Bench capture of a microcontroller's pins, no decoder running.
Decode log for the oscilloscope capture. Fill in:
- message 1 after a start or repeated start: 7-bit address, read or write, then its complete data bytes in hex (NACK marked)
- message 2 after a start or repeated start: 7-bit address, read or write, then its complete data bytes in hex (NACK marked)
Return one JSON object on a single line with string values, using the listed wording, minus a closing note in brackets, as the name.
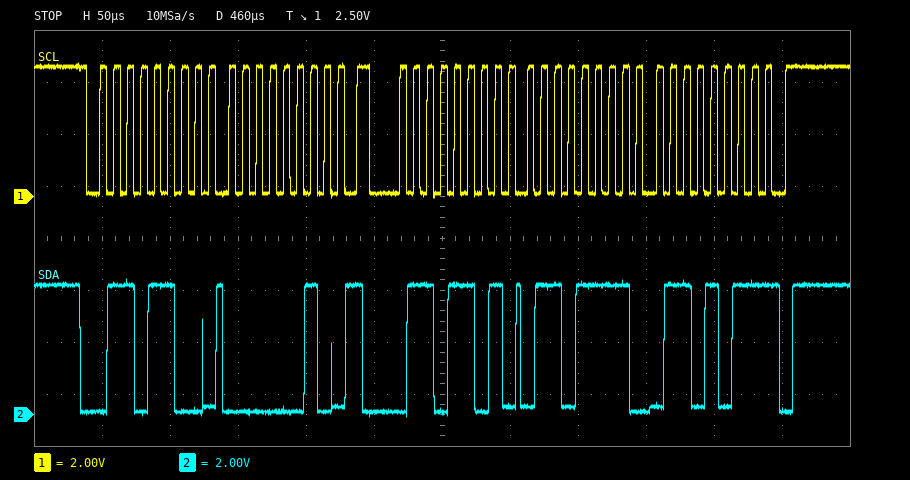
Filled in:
{"message 1 after a start or repeated start: 7-bit address, read or write, then its complete data bytes in hex": "0x36 write: 02", "message 2 after a start or repeated start: 7-bit address, read or write, then its complete data bytes in hex": "0x36 read: 6F 6B NACK"}
